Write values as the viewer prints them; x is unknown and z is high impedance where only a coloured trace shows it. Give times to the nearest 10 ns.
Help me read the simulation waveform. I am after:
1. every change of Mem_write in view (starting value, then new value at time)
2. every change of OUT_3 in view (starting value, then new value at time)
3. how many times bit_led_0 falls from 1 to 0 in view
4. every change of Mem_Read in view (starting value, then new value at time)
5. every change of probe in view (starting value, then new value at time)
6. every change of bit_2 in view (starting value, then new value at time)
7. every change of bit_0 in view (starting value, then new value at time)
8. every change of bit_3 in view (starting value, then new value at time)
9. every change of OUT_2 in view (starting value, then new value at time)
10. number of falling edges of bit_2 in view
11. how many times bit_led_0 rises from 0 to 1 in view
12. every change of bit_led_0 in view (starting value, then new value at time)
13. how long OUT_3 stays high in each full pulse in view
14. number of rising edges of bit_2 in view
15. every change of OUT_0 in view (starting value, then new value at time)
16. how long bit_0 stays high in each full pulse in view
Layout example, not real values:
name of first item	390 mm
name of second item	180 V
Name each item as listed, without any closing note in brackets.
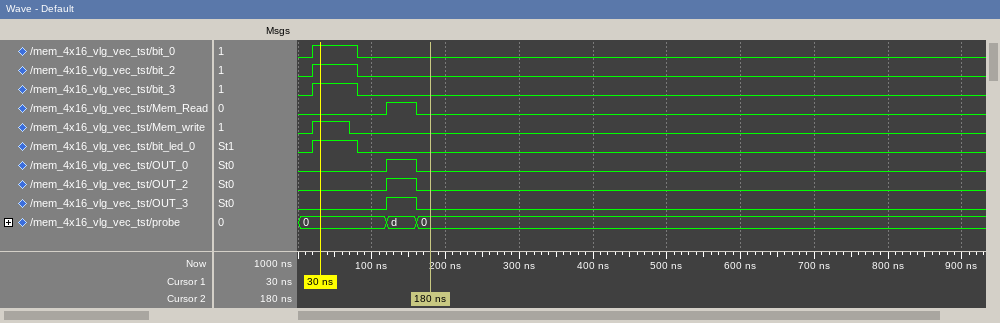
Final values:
every change of Mem_write in view	0, 1 at 20 ns, 0 at 70 ns
every change of OUT_3 in view	0, 1 at 120 ns, 0 at 160 ns
how many times bit_led_0 falls from 1 to 0 in view	1
every change of Mem_Read in view	0, 1 at 120 ns, 0 at 160 ns
every change of probe in view	0, d at 120 ns, 0 at 160 ns
every change of bit_2 in view	0, 1 at 20 ns, 0 at 80 ns
every change of bit_0 in view	0, 1 at 20 ns, 0 at 80 ns
every change of bit_3 in view	0, 1 at 20 ns, 0 at 80 ns
every change of OUT_2 in view	0, 1 at 120 ns, 0 at 160 ns
number of falling edges of bit_2 in view	1
how many times bit_led_0 rises from 0 to 1 in view	1
every change of bit_led_0 in view	0, 1 at 20 ns, 0 at 80 ns
how long OUT_3 stays high in each full pulse in view	40 ns
number of rising edges of bit_2 in view	1
every change of OUT_0 in view	0, 1 at 120 ns, 0 at 160 ns
how long bit_0 stays high in each full pulse in view	60 ns
